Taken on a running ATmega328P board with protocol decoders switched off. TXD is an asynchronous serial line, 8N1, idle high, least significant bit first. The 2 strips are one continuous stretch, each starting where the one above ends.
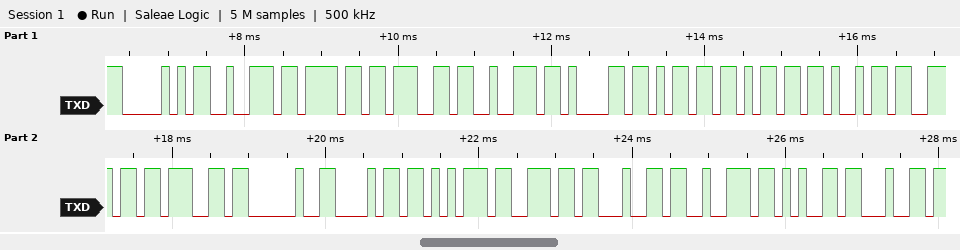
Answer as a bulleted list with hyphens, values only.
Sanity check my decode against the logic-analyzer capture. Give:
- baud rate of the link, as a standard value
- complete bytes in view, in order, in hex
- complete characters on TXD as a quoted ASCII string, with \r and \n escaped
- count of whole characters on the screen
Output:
- 9600 baud
- 50 72 6F 67 72 61 6D 6D 69 6E 67 20 68 75 6E 64 72 65 64
- "Programming hundred"
- 19
